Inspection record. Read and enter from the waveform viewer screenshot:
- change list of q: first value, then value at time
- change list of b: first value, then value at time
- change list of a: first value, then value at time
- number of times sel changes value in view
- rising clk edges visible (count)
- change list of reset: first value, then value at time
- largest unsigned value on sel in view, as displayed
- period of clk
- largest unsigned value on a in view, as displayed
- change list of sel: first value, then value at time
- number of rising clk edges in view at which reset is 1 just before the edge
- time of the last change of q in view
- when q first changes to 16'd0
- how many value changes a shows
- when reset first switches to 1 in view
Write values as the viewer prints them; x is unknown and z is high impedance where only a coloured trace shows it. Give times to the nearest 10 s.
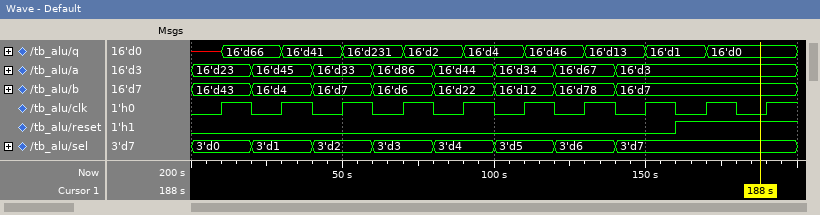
x, 16'd66 at 10 s, 16'd41 at 30 s, 16'd231 at 50 s, 16'd2 at 70 s, 16'd4 at 90 s, 16'd46 at 110 s, 16'd13 at 130 s, 16'd1 at 150 s, 16'd0 at 170 s
16'd43, 16'd4 at 20 s, 16'd7 at 40 s, 16'd6 at 60 s, 16'd22 at 80 s, 16'd12 at 100 s, 16'd78 at 120 s, 16'd7 at 140 s
16'd23, 16'd45 at 20 s, 16'd33 at 40 s, 16'd86 at 60 s, 16'd44 at 80 s, 16'd34 at 100 s, 16'd67 at 120 s, 16'd3 at 140 s
7
10
0, 1 at 160 s
3'd7
20 s
16'd86
3'd0, 3'd1 at 20 s, 3'd2 at 40 s, 3'd3 at 60 s, 3'd4 at 80 s, 3'd5 at 100 s, 3'd6 at 120 s, 3'd7 at 140 s
2
170 s
170 s
7
160 s
